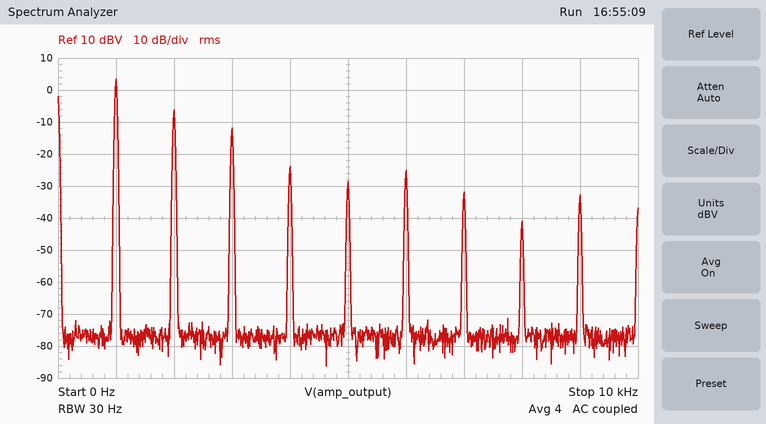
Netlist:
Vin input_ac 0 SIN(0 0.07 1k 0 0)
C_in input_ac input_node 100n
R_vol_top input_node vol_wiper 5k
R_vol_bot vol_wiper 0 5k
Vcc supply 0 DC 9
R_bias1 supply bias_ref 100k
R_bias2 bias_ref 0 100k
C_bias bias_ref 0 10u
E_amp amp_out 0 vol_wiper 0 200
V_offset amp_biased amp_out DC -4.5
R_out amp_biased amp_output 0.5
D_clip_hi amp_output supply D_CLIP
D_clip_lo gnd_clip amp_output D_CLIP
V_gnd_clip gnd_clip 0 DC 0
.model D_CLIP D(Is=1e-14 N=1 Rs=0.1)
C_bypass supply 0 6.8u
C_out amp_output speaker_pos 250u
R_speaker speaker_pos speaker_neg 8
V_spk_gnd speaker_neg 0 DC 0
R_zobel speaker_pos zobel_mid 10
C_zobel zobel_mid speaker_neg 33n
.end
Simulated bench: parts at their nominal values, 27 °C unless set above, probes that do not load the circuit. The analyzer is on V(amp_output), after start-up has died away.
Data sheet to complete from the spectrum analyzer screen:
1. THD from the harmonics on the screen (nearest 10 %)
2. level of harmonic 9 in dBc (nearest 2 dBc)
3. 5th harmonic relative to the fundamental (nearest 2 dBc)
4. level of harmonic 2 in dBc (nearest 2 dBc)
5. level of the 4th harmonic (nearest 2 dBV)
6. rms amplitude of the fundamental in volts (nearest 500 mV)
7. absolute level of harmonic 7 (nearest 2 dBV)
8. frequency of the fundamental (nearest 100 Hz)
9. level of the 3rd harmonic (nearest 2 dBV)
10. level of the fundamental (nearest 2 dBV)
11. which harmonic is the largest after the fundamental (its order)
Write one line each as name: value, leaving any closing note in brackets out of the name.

THD from the harmonics on the screen: 40 %
level of harmonic 9 in dBc: -36 dBc
5th harmonic relative to the fundamental: -32 dBc
level of harmonic 2 in dBc: -10 dBc
level of the 4th harmonic: -24 dBV
rms amplitude of the fundamental in volts: 1.5 V
absolute level of harmonic 7: -32 dBV
frequency of the fundamental: 1.0 kHz
level of the 3rd harmonic: -12 dBV
level of the fundamental: 4 dBV
which harmonic is the largest after the fundamental: 2
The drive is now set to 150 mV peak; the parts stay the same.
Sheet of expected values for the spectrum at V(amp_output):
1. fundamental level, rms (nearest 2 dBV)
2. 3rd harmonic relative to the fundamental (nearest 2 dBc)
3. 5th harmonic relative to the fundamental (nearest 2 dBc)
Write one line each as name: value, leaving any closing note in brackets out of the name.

fundamental level, rms: 14 dBV
3rd harmonic relative to the fundamental: -22 dBc
5th harmonic relative to the fundamental: -28 dBc
